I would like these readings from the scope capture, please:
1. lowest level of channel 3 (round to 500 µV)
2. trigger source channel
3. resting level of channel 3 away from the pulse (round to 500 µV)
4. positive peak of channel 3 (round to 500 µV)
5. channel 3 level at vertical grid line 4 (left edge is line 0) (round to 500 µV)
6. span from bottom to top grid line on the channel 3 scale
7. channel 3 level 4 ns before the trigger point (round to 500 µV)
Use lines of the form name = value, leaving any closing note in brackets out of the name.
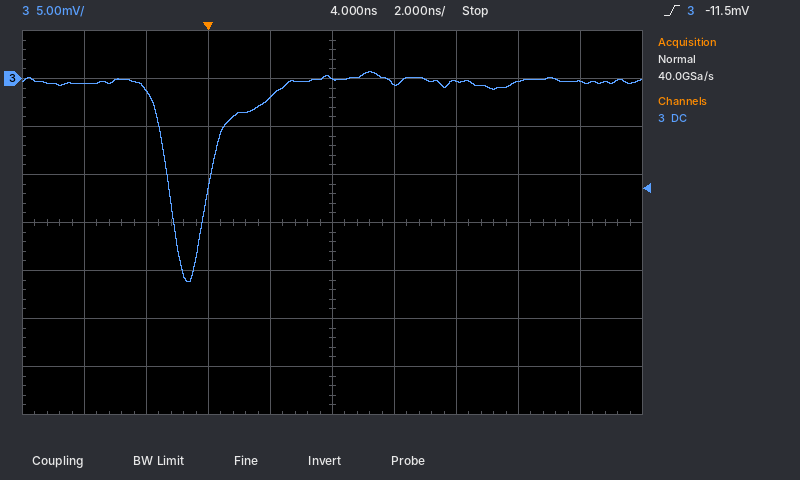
lowest level of channel 3 = -21.0 mV
trigger source channel = channel 3
resting level of channel 3 away from the pulse = -500 µV
positive peak of channel 3 = 500 µV
channel 3 level at vertical grid line 4 (left edge is line 0) = -2.0 mV
span from bottom to top grid line on the channel 3 scale = 40 mV
channel 3 level 4 ns before the trigger point = -500 µV
